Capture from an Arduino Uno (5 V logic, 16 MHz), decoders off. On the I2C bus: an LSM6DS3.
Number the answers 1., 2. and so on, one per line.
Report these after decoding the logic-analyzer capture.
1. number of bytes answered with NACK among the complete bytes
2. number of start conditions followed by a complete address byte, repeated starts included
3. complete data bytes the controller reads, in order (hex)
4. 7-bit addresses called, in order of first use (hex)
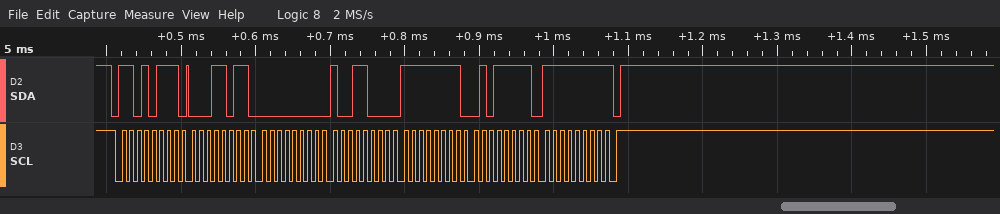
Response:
1. 1
2. 1
3. 1B 00 98 FF 5F FF
4. 0x6B
